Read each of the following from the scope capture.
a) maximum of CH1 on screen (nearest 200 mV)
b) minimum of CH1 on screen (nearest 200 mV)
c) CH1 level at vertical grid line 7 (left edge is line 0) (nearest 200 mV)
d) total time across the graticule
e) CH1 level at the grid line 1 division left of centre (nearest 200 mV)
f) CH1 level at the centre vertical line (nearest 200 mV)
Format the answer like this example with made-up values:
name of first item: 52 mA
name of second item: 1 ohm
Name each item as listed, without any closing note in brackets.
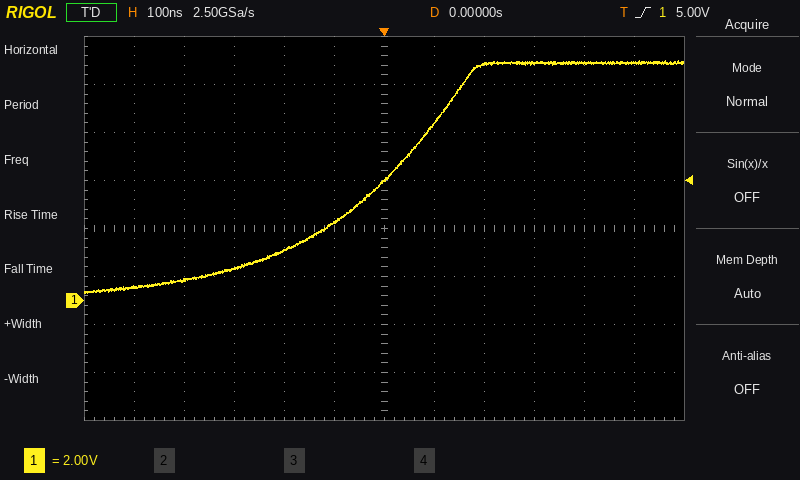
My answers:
maximum of CH1 on screen: 10.0 V
minimum of CH1 on screen: 200 mV
CH1 level at vertical grid line 7 (left edge is line 0): 7.4 V
total time across the graticule: 1.2 µs
CH1 level at the grid line 1 division left of centre: 3.2 V
CH1 level at the centre vertical line: 5.0 V
